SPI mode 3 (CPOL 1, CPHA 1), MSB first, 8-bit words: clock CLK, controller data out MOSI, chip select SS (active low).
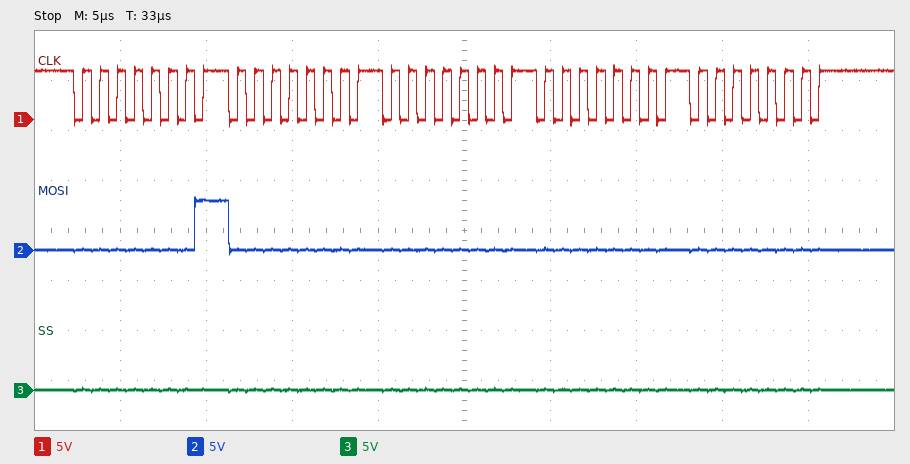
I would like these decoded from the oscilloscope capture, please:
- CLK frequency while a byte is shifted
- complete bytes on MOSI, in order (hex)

1 MHz
0x01 0x00 0x00 0x00 0x00
